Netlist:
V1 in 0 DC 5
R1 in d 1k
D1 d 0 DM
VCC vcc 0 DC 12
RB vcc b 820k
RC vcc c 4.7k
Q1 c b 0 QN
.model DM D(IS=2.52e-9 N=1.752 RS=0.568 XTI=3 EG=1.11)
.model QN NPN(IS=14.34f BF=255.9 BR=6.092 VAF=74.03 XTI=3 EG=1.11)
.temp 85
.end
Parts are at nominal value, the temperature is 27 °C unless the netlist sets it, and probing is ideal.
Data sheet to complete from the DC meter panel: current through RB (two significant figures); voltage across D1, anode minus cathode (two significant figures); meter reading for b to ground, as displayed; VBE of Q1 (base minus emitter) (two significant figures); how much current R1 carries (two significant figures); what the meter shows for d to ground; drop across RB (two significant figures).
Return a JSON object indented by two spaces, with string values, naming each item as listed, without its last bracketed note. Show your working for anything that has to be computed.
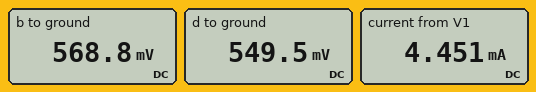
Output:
{
  "current through RB": "(12 V - 568.8 mV) / 820 kΩ = 14 µA",
  "voltage across D1, anode minus cathode": "549.5 mV = 550 mV",
  "meter reading for b to ground, as displayed": "568.8 mV",
  "VBE of Q1 (base minus emitter)": "568.8 mV = 570 mV",
  "how much current R1 carries": "(5 V - 549.5 mV) / 1 kΩ = 4.5 mA",
  "what the meter shows for d to ground": "549.5 mV",
  "drop across RB": "12 V - 568.8 mV = 11 V"
}
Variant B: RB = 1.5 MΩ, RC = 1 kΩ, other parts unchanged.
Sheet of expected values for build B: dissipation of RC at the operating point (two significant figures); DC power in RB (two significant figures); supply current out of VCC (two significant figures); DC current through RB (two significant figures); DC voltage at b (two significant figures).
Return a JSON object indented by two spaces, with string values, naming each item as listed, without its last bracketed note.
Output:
{
  "dissipation of RC at the operating point": "4.8 mW",
  "DC power in RB": "87 µW",
  "supply current out of VCC": "2.2 mA",
  "DC current through RB": "7.6 µA",
  "DC voltage at b": "560 mV"
}
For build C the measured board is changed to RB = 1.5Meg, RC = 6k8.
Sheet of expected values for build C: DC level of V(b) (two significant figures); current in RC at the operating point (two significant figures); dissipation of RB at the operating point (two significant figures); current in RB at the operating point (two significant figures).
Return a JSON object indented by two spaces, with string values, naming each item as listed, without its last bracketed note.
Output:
{
  "DC level of V(b)": "560 mV",
  "current in RC at the operating point": "1.7 mA",
  "dissipation of RB at the operating point": "87 µW",
  "current in RB at the operating point": "7.6 µA"
}
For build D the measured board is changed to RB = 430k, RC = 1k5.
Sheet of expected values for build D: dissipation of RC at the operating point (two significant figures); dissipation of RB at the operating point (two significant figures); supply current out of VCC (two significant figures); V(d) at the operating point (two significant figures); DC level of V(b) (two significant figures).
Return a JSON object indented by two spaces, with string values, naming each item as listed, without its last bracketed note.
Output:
{
  "dissipation of RC at the operating point": "71 mW",
  "dissipation of RB at the operating point": "300 µW",
  "supply current out of VCC": "6.9 mA",
  "V(d) at the operating point": "550 mV",
  "DC level of V(b)": "600 mV"
}
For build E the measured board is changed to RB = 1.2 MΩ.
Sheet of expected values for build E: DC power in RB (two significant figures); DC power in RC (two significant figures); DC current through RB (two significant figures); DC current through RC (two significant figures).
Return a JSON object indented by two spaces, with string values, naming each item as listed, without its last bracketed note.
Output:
{
  "DC power in RB": "110 µW",
  "DC power in RC": "28 mW",
  "DC current through RB": "9.5 µA",
  "DC current through RC": "2.4 mA"
}
